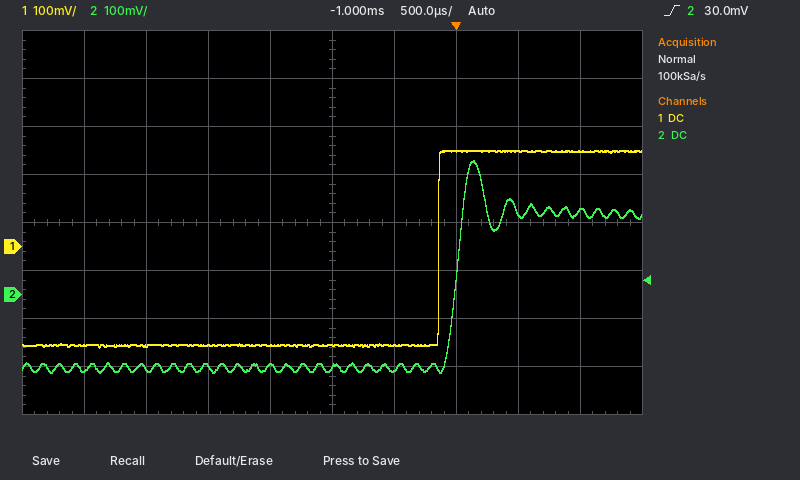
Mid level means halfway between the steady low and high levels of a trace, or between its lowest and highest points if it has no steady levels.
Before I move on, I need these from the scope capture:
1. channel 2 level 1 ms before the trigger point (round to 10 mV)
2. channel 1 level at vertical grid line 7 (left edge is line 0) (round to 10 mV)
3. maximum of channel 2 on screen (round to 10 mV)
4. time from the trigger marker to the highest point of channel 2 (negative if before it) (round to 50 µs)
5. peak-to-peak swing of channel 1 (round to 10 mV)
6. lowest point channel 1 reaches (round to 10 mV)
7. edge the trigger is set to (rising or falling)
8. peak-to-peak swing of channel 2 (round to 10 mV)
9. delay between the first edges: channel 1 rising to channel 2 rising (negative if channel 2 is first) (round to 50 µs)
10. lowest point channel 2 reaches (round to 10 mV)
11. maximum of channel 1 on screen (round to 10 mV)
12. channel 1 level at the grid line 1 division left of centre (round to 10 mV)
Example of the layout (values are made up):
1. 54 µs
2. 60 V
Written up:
1. -150 mV
2. 200 mV
3. 280 mV
4. +150 µs
5. 410 mV
6. -210 mV
7. rising
8. 440 mV
9. +150 µs
10. -160 mV
11. 200 mV
12. -210 mV
